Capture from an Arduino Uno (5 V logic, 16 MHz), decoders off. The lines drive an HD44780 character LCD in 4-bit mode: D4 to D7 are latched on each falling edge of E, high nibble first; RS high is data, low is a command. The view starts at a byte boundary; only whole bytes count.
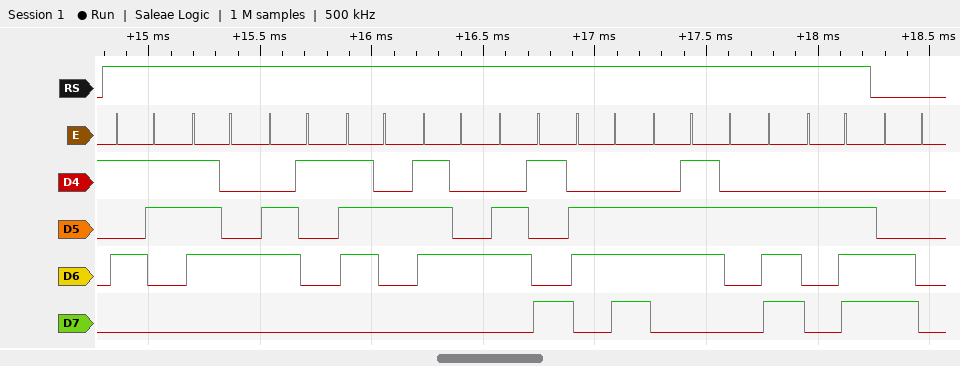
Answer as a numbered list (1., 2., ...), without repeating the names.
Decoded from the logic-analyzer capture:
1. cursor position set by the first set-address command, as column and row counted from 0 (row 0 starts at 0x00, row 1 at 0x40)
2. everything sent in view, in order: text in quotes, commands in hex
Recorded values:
1. column 0, row 1
2. "Starting.." 0xC0
